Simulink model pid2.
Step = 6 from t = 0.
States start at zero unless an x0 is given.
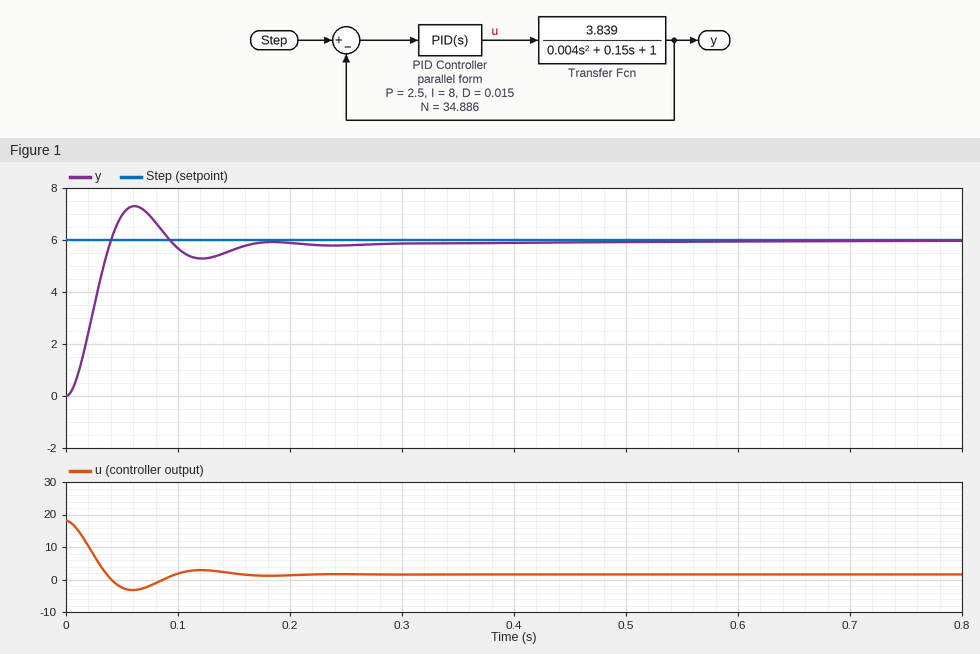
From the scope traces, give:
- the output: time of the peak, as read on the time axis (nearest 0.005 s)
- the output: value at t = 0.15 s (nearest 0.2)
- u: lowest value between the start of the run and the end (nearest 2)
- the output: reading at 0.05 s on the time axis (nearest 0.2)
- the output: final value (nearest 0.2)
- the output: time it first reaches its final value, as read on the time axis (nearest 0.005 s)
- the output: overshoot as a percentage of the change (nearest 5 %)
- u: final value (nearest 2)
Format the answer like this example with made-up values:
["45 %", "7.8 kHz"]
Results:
["0.060 s", "5.6", "-4", "7.0", "6.0", "0.040 s", "20 %", "2"]
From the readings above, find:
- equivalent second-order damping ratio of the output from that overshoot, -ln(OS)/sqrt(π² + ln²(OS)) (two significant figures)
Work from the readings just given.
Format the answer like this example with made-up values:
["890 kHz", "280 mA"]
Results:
["0.46"]
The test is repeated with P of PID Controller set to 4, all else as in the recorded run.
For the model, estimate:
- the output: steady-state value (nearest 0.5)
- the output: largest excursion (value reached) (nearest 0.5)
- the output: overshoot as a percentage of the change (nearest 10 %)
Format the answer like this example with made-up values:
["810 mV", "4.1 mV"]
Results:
["6.0", "8.0", "30 %"]
